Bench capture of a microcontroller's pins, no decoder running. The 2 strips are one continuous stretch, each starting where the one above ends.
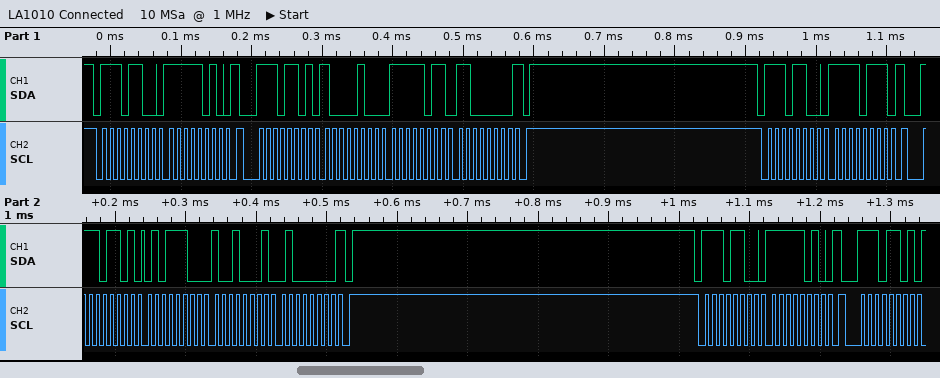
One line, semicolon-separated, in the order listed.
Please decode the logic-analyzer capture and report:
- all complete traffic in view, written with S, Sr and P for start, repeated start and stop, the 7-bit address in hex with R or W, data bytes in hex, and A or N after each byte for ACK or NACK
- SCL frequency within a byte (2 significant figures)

S 76W A FA A Sr 76R A 84 A FB A C0 N P S 76W A F7 A Sr 76R A 5C A 91 A 40 N P S 76W A FA A Sr 76R A; 100 kHz
